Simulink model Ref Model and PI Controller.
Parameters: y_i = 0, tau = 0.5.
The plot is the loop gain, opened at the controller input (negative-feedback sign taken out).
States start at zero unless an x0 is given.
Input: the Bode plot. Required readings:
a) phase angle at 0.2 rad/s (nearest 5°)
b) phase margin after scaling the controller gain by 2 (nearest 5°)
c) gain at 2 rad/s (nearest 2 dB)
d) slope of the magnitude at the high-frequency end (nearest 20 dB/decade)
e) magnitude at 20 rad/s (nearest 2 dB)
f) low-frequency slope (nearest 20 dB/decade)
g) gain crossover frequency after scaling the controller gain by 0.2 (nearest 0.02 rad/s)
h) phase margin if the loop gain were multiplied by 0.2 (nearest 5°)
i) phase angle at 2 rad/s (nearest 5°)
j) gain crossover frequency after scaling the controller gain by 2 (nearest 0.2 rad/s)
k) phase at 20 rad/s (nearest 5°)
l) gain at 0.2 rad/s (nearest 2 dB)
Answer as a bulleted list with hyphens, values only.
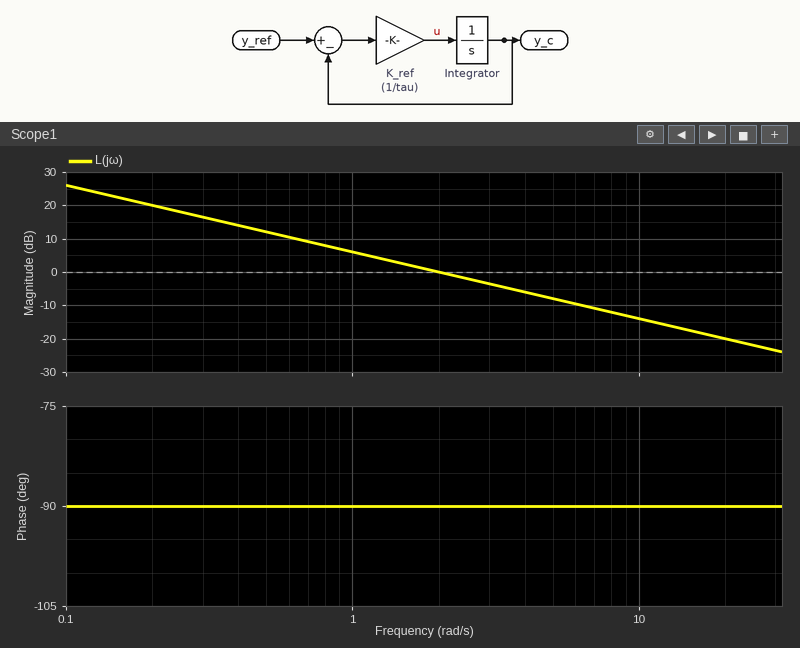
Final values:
- -90°
- 90°
- 0 dB
- -20 dB/decade
- -20 dB
- -20 dB/decade
- 0.40 rad/s
- 90°
- -90°
- 4.0 rad/s
- -90°
- 20 dB
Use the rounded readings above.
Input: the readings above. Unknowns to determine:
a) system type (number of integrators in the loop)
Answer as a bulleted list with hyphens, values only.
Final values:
- 1
